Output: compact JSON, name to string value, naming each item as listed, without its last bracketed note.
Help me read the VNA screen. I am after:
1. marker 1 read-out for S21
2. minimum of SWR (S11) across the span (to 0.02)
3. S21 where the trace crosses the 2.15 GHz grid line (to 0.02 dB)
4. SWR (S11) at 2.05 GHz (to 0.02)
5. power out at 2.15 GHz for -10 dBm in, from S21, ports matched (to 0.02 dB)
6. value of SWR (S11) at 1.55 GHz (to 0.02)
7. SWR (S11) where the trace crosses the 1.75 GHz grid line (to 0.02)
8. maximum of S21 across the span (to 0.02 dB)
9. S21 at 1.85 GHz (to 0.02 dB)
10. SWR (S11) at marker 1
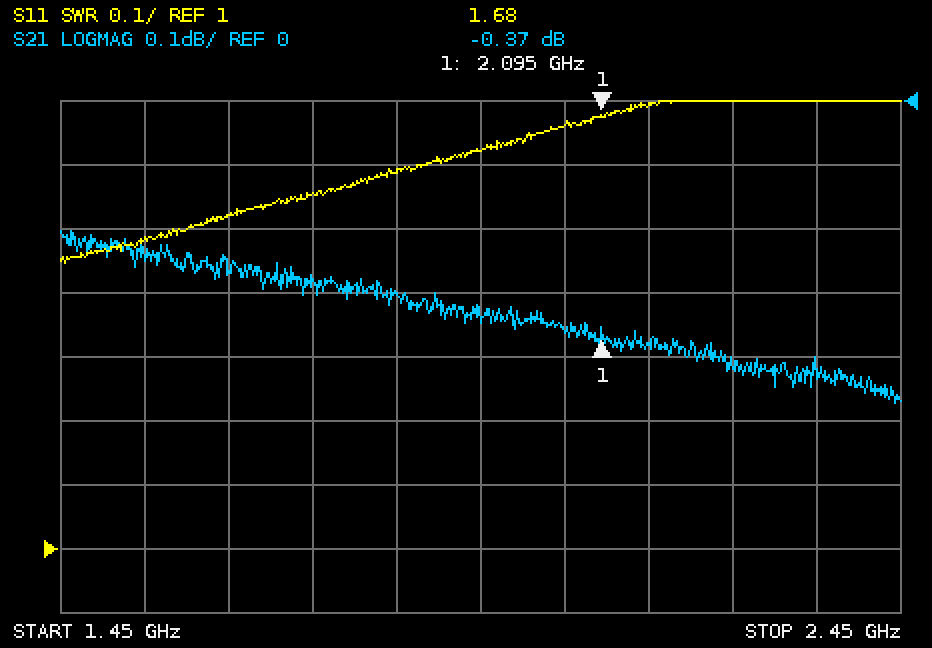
{"marker 1 read-out for S21": "-0.37 dB", "minimum of SWR (S11) across the span": "1.44", "S21 where the trace crosses the 2.15 GHz grid line": "-0.38 dB", "SWR (S11) at 2.05 GHz": "1.66", "power out at 2.15 GHz for -10 dBm in, from S21, ports matched": "-10.38 dBm", "value of SWR (S11) at 1.55 GHz": "1.48", "SWR (S11) where the trace crosses the 1.75 GHz grid line": "1.56", "maximum of S21 across the span": "-0.20 dB", "S21 at 1.85 GHz": "-0.30 dB", "SWR (S11) at marker 1": "1.68"}
